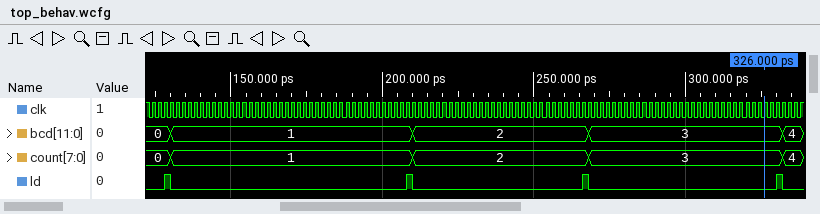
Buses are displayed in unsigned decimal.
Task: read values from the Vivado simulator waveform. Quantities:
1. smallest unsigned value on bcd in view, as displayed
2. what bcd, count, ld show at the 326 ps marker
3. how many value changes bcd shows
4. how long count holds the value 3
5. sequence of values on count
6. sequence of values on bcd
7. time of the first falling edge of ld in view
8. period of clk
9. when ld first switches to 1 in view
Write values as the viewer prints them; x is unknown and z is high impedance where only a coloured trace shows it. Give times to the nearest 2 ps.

0
bcd=3, count=3, ld=0
4
64 ps
0, 1, 2, 3, 4
0, 1, 2, 3, 4
130 ps
2 ps
128 ps
